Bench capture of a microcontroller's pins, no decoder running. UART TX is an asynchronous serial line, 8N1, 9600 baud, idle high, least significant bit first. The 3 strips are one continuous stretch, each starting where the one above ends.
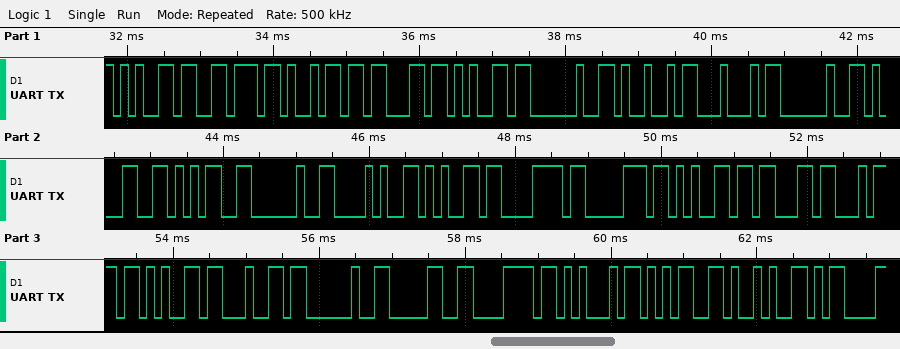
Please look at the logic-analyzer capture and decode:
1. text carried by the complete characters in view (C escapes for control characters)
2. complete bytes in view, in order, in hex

"evice ID 15 (expected 0xE5)\r"
0x65 0x76 0x69 0x63 0x65 0x20 0x49 0x44 0x20 0x31 0x35 0x20 0x28 0x65 0x78 0x70 0x65 0x63 0x74 0x65 0x64 0x20 0x30 0x78 0x45 0x35 0x29 0x0D
